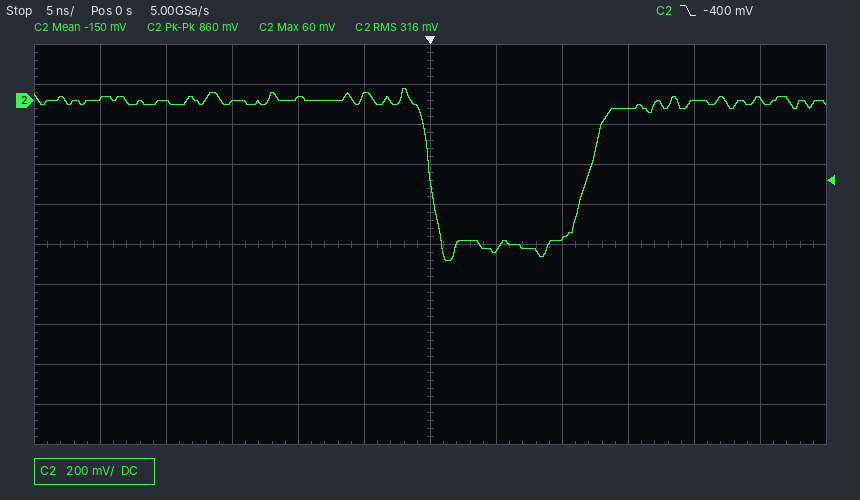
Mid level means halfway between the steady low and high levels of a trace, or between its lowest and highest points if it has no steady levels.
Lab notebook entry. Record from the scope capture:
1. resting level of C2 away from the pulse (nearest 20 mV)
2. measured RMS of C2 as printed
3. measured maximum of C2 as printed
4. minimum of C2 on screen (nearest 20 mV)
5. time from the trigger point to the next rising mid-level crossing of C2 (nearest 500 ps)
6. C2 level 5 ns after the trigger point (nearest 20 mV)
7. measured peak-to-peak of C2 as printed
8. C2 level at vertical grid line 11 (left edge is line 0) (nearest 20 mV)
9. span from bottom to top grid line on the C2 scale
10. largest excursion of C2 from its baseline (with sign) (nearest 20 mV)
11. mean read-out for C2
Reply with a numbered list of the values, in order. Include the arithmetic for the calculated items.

1. 0 mV
2. 316 mV
3. 60 mV
4. -800 mV
5. 12.0 ns
6. -740 mV
7. 860 mV
8. 0 mV
9. 2 V
10. -800 mV − (0 mV) = -800 mV
11. -150 mV
